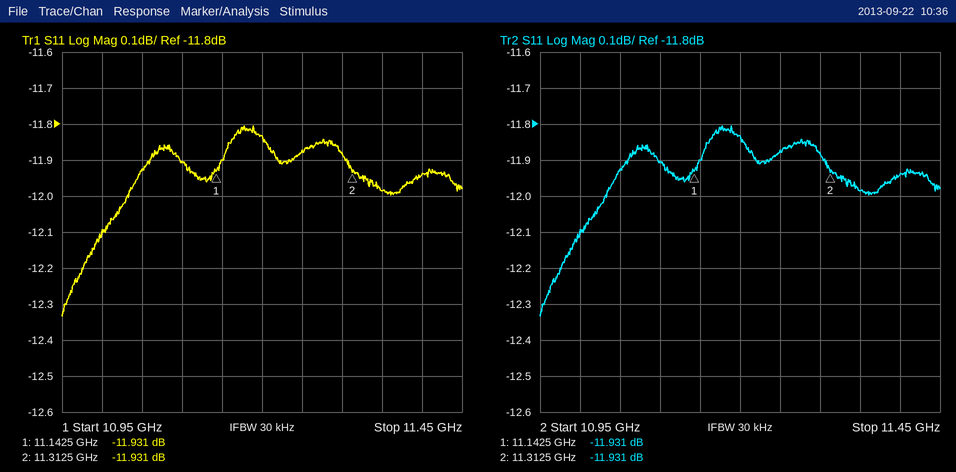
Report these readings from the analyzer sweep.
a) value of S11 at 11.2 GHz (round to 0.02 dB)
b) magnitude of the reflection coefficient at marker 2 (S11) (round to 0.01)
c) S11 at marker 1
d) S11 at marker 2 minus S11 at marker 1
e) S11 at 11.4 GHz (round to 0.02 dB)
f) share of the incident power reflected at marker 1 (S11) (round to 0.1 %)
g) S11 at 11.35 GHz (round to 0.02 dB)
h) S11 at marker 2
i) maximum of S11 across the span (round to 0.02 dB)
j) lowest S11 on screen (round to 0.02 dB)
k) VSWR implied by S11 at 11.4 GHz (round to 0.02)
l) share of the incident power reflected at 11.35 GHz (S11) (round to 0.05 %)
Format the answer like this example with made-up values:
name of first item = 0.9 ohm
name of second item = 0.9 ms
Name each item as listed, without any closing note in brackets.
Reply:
value of S11 at 11.2 GHz = -11.84 dB
magnitude of the reflection coefficient at marker 2 (S11) = 0.25
S11 at marker 1 = -11.931 dB
S11 at marker 2 minus S11 at marker 1 = 0.000 dB
S11 at 11.4 GHz = -11.94 dB
share of the incident power reflected at marker 1 (S11) = 6.4 %
S11 at 11.35 GHz = -11.98 dB
S11 at marker 2 = -11.931 dB
maximum of S11 across the span = -11.80 dB
lowest S11 on screen = -12.34 dB
VSWR implied by S11 at 11.4 GHz = 1.68
share of the incident power reflected at 11.35 GHz (S11) = 6.35 %
